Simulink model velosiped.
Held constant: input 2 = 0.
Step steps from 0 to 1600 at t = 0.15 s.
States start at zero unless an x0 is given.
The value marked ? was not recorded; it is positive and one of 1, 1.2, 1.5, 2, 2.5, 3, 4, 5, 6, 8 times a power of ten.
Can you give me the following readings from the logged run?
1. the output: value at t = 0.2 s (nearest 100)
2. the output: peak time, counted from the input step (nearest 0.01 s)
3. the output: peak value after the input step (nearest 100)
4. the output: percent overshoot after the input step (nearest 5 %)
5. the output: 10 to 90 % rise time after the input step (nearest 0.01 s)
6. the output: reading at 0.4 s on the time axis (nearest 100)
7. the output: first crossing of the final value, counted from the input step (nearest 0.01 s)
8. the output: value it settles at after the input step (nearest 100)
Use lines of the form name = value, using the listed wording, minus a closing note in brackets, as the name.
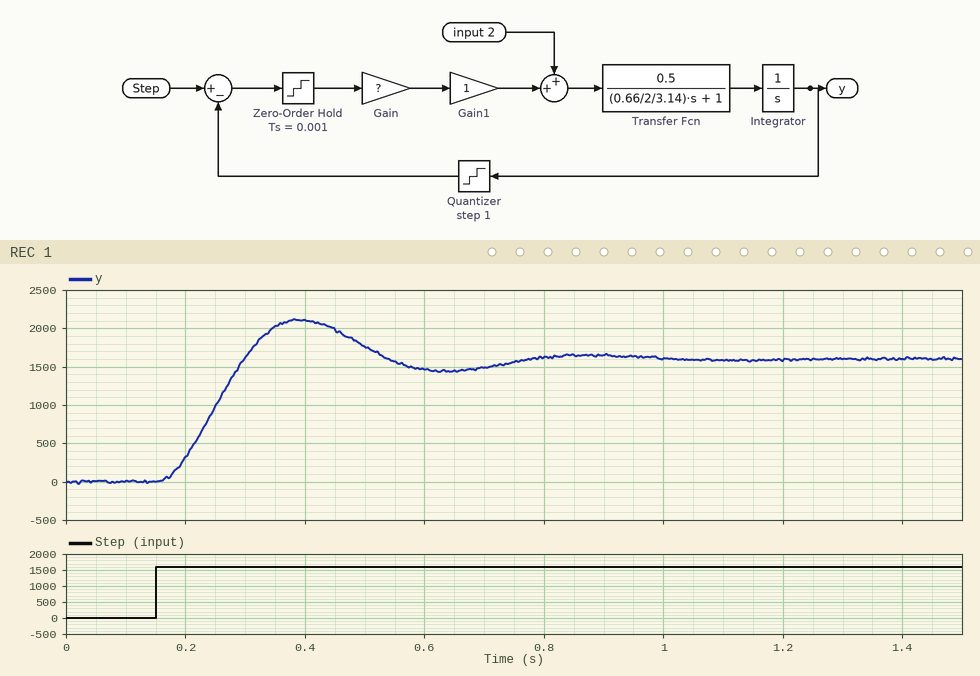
the output: value at t = 0.2 s = 300
the output: peak time, counted from the input step = 0.24 s
the output: peak value after the input step = 2100
the output: percent overshoot after the input step = 30 %
the output: 10 to 90 % rise time after the input step = 0.10 s
the output: reading at 0.4 s on the time axis = 2100
the output: first crossing of the final value, counted from the input step = 0.15 s
the output: value it settles at after the input step = 1600
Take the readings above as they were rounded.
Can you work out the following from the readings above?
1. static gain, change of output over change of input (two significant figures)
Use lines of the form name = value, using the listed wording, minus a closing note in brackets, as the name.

static gain, change of output over change of input = 1.0
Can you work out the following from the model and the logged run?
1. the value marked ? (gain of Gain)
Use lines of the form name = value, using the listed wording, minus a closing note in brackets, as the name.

the value marked ? = 40
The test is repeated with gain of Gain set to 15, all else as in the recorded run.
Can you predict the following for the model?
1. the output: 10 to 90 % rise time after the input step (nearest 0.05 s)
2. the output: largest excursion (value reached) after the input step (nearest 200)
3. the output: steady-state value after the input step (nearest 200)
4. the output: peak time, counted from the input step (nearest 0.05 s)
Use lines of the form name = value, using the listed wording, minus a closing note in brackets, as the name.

the output: 10 to 90 % rise time after the input step = 0.20 s
the output: largest excursion (value reached) after the input step = 1800
the output: steady-state value after the input step = 1600
the output: peak time, counted from the input step = 0.45 s
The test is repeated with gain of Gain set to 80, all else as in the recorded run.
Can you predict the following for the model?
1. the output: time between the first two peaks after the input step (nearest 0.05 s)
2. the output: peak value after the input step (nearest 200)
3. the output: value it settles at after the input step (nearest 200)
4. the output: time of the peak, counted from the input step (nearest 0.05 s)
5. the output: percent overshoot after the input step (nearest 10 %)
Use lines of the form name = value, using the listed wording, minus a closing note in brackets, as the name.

the output: time between the first two peaks after the input step = 0.35 s
the output: peak value after the input step = 2400
the output: value it settles at after the input step = 1600
the output: time of the peak, counted from the input step = 0.15 s
the output: percent overshoot after the input step = 50 %
